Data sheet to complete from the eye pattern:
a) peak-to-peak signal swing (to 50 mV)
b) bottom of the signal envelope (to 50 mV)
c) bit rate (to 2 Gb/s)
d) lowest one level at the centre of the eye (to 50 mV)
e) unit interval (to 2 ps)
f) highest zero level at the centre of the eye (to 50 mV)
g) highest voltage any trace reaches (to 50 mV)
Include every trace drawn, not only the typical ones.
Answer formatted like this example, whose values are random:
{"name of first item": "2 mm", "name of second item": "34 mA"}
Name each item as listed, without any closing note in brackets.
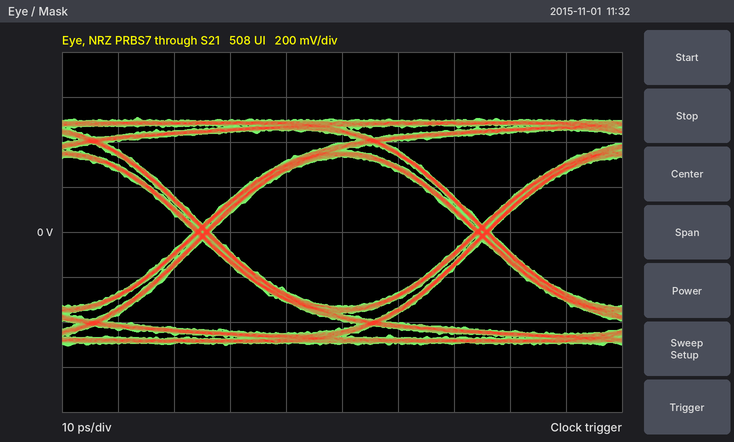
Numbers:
{"peak-to-peak signal swing": "1.00 V", "bottom of the signal envelope": "-500 mV", "bit rate": "20 Gb/s", "lowest one level at the centre of the eye": "350 mV", "unit interval": "50 ps", "highest zero level at the centre of the eye": "-350 mV", "highest voltage any trace reaches": "500 mV"}
